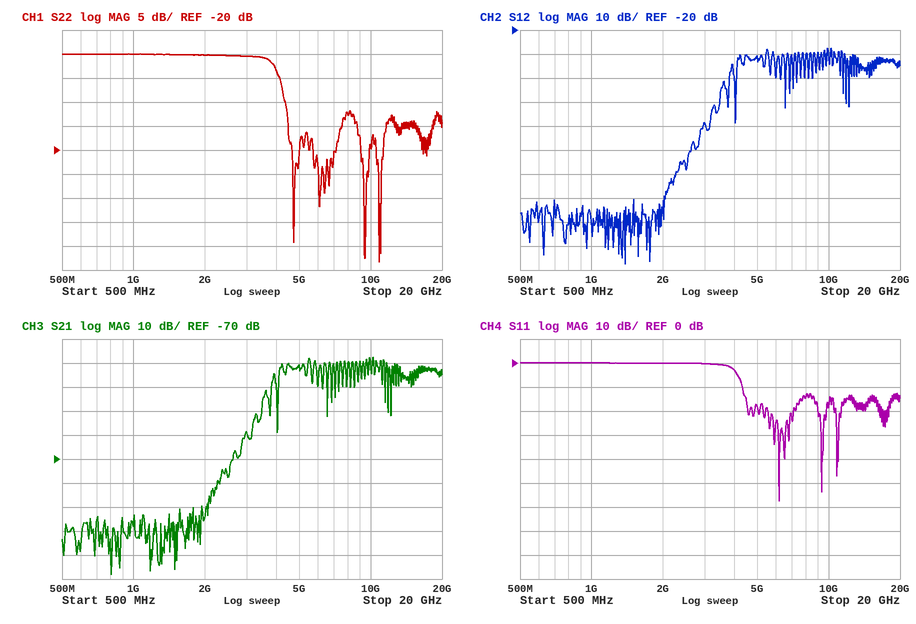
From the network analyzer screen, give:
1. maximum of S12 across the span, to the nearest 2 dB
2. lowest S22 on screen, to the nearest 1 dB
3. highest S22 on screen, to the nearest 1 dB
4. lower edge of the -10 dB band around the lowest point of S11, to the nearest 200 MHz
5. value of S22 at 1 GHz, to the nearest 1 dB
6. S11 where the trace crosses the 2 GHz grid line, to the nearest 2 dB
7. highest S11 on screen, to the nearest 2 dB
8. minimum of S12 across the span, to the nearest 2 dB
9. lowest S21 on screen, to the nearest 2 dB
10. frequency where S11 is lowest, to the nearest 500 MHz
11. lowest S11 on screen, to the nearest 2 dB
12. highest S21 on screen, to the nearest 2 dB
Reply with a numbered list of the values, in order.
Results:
1. -28 dB
2. -43 dB
3. 0 dB
4. 4.4 GHz
5. 0 dB
6. 0 dB
7. 0 dB
8. -118 dB
9. -118 dB
10. 6.0 GHz
11. -58 dB
12. -28 dB
